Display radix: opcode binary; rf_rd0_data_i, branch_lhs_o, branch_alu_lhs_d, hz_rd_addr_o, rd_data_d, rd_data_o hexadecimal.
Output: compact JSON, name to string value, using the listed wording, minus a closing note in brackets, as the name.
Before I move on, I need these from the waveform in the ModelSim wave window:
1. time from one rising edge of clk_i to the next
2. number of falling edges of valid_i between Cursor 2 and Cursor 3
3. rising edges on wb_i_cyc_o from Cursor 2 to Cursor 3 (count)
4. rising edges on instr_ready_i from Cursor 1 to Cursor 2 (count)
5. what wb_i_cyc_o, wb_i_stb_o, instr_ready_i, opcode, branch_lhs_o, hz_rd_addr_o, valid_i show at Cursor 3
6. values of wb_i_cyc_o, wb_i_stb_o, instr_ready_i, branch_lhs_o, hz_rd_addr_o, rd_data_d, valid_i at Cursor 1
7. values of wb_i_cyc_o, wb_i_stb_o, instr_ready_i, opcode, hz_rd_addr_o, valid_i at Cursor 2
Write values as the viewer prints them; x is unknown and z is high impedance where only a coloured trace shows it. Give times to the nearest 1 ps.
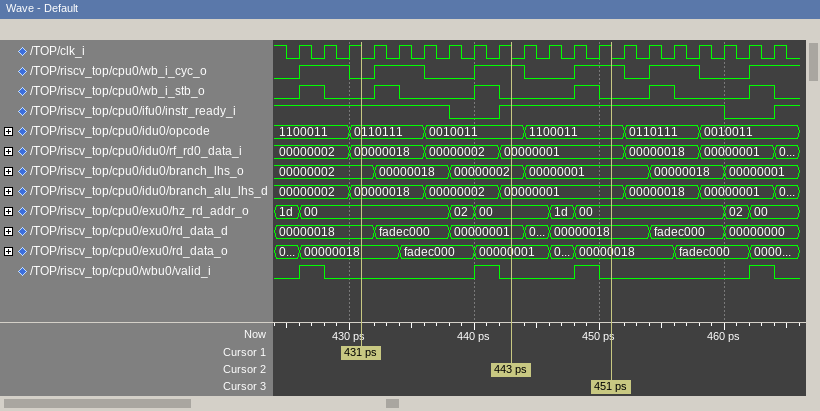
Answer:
{"time from one rising edge of clk_i to the next": "2 ps", "number of falling edges of valid_i between Cursor 2 and Cursor 3": "1", "rising edges on wb_i_cyc_o from Cursor 2 to Cursor 3": "1", "rising edges on instr_ready_i from Cursor 1 to Cursor 2": "1", "what wb_i_cyc_o, wb_i_stb_o, instr_ready_i, opcode, branch_lhs_o, hz_rd_addr_o, valid_i show at Cursor 3": "wb_i_cyc_o=1, wb_i_stb_o=0, instr_ready_i=1, opcode=1100011, branch_lhs_o=00000001, hz_rd_addr_o=00, valid_i=0", "values of wb_i_cyc_o, wb_i_stb_o, instr_ready_i, branch_lhs_o, hz_rd_addr_o, rd_data_d, valid_i at Cursor 1": "wb_i_cyc_o=0, wb_i_stb_o=0, instr_ready_i=1, branch_lhs_o=00000002, hz_rd_addr_o=00, rd_data_d=00000018, valid_i=0", "values of wb_i_cyc_o, wb_i_stb_o, instr_ready_i, opcode, hz_rd_addr_o, valid_i at Cursor 2": "wb_i_cyc_o=1, wb_i_stb_o=0, instr_ready_i=1, opcode=0010011, hz_rd_addr_o=00, valid_i=0"}
